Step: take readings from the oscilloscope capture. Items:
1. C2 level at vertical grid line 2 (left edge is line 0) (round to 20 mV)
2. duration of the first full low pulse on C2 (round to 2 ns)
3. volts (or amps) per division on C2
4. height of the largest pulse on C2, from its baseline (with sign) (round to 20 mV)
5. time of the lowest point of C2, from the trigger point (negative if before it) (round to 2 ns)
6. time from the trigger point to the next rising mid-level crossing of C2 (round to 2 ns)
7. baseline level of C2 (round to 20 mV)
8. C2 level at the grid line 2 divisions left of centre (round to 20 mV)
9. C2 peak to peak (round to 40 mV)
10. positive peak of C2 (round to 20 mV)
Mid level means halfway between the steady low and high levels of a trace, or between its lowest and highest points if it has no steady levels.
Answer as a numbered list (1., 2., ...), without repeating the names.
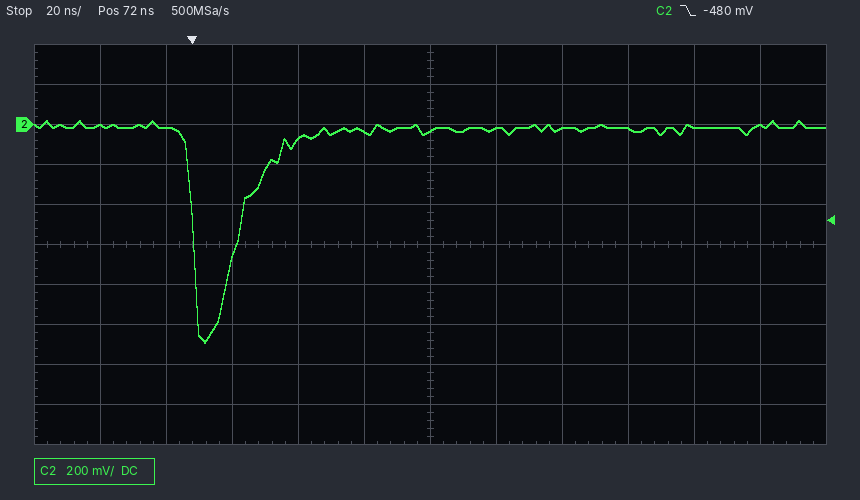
1. -20 mV
2. 14 ns
3. 200 mV
4. -1.08 V
5. +4 ns
6. 14 ns
7. -20 mV
8. -80 mV
9. 1.12 V
10. 20 mV
